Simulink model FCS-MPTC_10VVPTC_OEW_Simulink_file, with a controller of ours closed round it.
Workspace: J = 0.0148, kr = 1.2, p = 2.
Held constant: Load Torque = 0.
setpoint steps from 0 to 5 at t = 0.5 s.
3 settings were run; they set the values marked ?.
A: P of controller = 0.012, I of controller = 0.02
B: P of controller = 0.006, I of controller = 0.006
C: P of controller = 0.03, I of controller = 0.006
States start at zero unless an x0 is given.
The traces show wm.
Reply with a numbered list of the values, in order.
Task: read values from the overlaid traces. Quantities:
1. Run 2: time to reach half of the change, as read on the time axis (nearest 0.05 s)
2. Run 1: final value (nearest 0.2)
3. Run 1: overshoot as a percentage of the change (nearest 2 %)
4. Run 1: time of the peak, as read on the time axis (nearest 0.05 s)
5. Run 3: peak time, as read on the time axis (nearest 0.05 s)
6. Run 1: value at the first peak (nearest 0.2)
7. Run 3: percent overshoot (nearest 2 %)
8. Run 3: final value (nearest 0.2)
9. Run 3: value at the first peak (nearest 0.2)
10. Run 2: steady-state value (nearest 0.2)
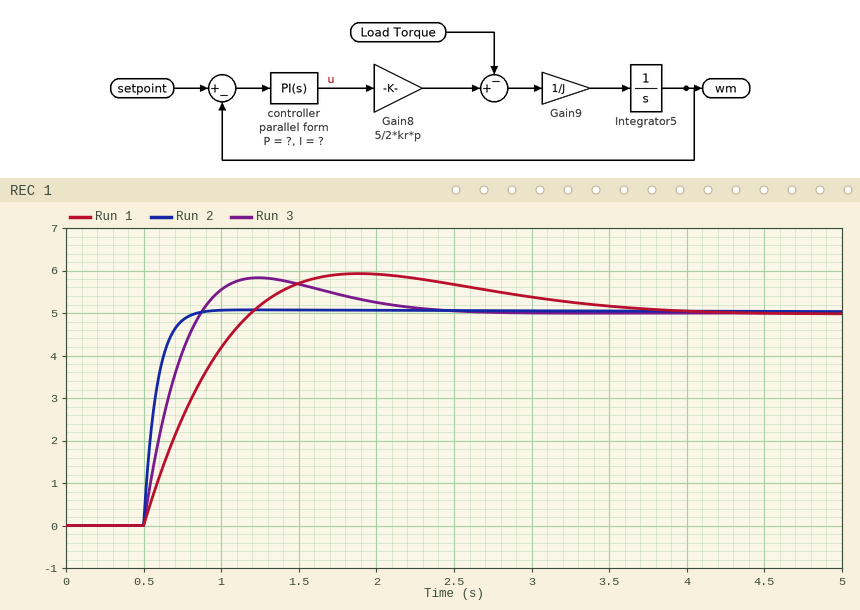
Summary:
1. 0.55 s
2. 5.0
3. 18 %
4. 1.90 s
5. 1.25 s
6. 6.0
7. 16 %
8. 5.0
9. 5.8
10. 5.0
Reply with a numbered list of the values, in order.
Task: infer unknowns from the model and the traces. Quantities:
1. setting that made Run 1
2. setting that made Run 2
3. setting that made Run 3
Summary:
1. B
2. C
3. A
